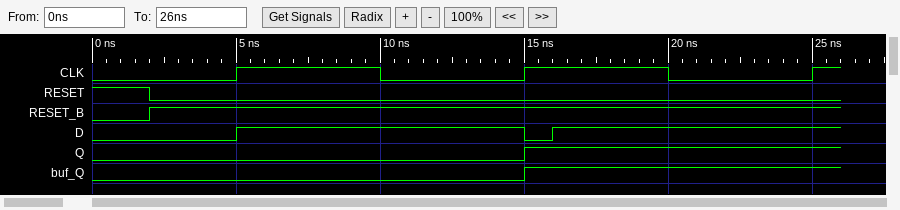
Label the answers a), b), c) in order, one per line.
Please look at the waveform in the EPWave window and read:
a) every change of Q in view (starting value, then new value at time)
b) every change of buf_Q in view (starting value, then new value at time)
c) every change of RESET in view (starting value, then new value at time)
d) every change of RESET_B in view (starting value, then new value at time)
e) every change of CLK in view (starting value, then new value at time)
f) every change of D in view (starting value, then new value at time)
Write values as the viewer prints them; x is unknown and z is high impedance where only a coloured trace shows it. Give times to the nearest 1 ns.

a) 0, 1 at 15 ns
b) 0, 1 at 15 ns
c) 1, 0 at 2 ns
d) 0, 1 at 2 ns
e) 0, 1 at 5 ns, 0 at 10 ns, 1 at 15 ns, 0 at 20 ns, 1 at 25 ns
f) 0, 1 at 5 ns, 0 at 15 ns, 1 at 16 ns
